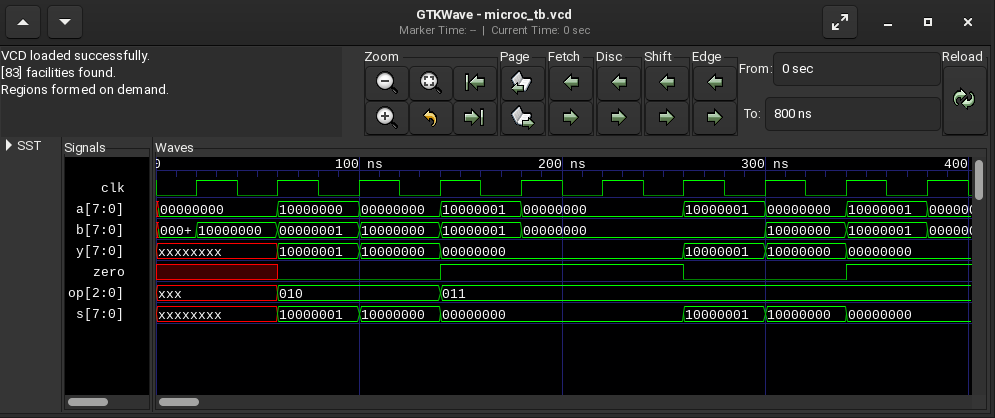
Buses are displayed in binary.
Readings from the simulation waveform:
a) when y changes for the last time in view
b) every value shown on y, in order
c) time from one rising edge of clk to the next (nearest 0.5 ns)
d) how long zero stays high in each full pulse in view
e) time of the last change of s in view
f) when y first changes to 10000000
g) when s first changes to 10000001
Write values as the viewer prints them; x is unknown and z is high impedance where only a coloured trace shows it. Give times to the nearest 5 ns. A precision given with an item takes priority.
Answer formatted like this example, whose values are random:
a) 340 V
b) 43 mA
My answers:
a) 340 ns
b) xxxxxxxx, 10000001, 10000000, 00000000, 10000001, 10000000, 00000000
c) 40 ns
d) 120 ns
e) 340 ns
f) 100 ns
g) 60 ns
